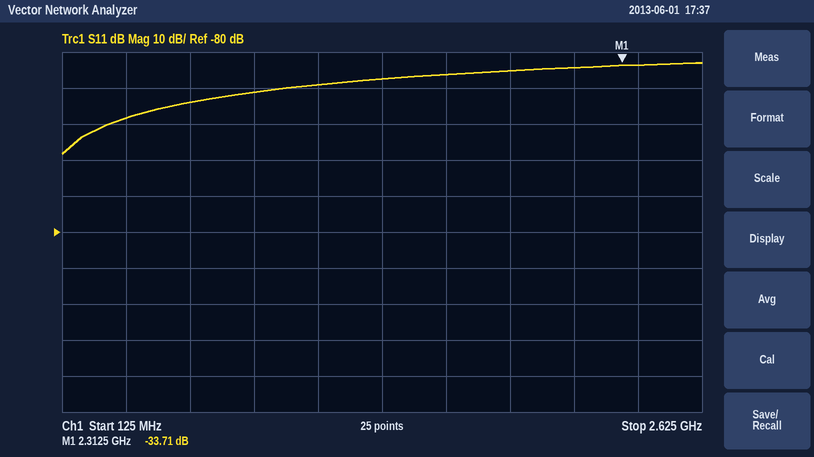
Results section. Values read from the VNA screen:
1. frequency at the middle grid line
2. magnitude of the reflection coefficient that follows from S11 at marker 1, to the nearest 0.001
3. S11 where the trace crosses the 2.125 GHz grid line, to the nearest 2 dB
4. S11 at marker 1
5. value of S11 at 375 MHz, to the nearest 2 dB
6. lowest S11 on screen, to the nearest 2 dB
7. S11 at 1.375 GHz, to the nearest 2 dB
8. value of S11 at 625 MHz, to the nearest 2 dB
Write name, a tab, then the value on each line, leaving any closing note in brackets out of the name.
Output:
frequency at the middle grid line	1.375 GHz
magnitude of the reflection coefficient that follows from S11 at marker 1, to the nearest 0.001	0.021
S11 where the trace crosses the 2.125 GHz grid line, to the nearest 2 dB	-34 dB
S11 at marker 1	-33.71 dB
value of S11 at 375 MHz, to the nearest 2 dB	-48 dB
lowest S11 on screen, to the nearest 2 dB	-58 dB
S11 at 1.375 GHz, to the nearest 2 dB	-38 dB
value of S11 at 625 MHz, to the nearest 2 dB	-44 dB
